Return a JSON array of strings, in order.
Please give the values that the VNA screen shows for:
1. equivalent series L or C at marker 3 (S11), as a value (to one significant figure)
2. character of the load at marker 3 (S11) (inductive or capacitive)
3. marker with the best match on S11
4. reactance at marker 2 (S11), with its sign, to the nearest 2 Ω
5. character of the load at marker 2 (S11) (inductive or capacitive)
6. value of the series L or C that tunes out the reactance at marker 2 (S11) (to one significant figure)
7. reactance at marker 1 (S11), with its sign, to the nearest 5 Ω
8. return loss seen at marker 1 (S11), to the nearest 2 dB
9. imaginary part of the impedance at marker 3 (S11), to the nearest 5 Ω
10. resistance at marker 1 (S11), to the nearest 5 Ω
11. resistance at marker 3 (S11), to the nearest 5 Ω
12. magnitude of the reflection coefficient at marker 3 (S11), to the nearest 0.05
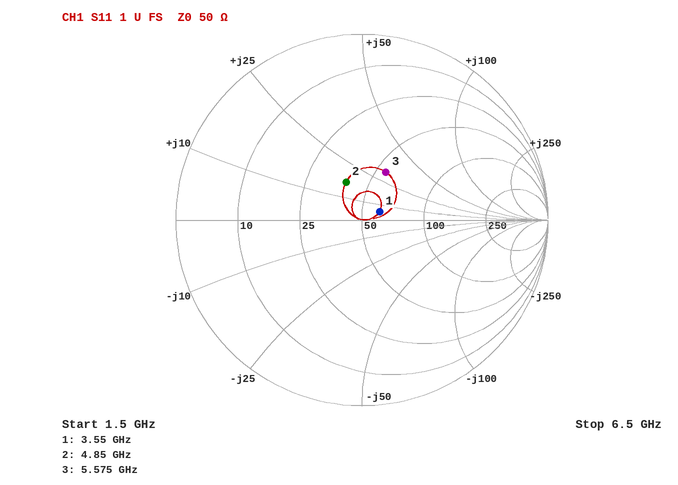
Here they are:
["900 pH", "inductive", "marker 1", "+16 Ω", "inductive", "2 pF", "+5 Ω", "20 dB", "+30 Ω", "60 Ω", "55 Ω", "0.30"]
